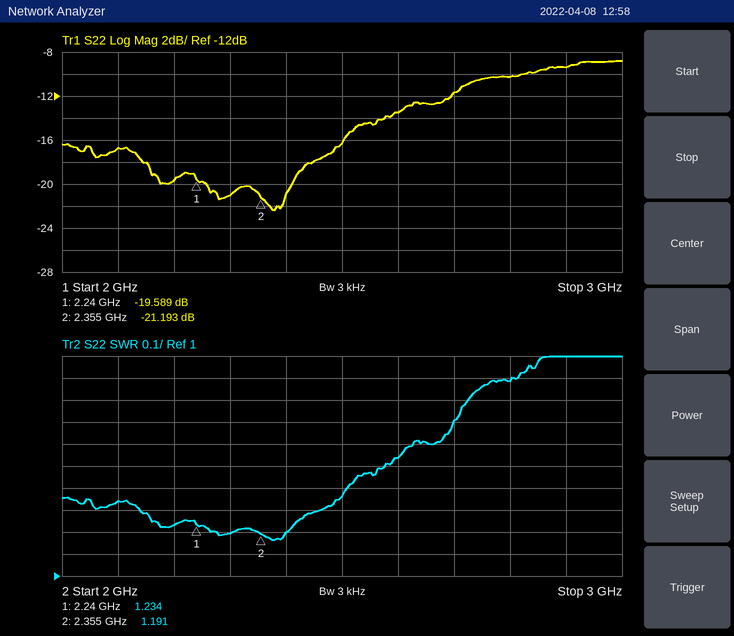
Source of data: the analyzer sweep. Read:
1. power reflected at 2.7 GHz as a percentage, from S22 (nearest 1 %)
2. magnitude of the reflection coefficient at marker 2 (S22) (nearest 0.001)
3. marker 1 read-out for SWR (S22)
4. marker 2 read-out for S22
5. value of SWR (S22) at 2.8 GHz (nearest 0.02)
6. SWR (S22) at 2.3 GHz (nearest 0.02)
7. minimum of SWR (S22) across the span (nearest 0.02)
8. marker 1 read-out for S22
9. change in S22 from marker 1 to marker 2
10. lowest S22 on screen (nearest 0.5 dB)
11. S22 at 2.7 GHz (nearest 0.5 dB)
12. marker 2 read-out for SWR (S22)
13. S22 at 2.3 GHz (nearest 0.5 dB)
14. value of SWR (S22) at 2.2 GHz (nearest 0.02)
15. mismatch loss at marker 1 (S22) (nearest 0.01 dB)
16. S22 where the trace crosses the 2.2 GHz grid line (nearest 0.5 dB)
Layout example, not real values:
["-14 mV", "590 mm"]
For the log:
["7 %", "0.087", "1.234", "-21.193 dB", "1.88", "1.20", "1.16", "-19.589 dB", "-1.604 dB", "-22.5 dB", "-11.5 dB", "1.191", "-21.0 dB", "1.24", "0.05 dB", "-19.5 dB"]
